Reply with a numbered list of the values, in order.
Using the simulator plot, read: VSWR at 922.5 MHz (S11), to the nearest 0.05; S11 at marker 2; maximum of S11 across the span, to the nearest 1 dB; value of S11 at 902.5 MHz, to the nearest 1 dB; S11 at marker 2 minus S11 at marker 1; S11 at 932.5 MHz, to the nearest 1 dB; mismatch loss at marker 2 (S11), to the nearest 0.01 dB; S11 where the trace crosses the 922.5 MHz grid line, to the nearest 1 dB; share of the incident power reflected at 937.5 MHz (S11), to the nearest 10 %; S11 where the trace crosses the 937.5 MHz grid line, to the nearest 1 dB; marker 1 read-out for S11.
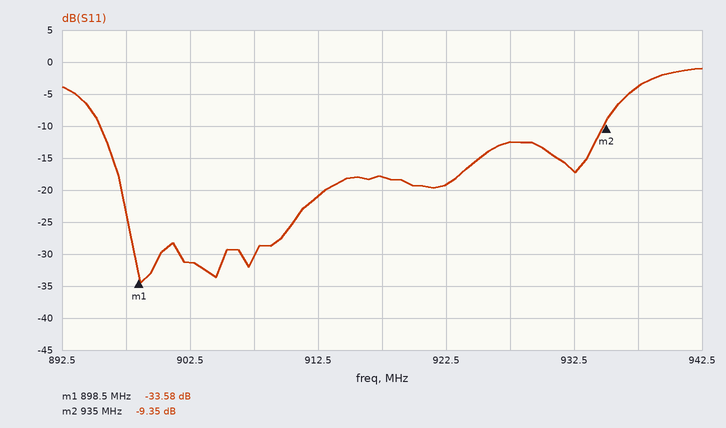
1. 1.25
2. -9.35 dB
3. -1 dB
4. -31 dB
5. 24.23 dB
6. -17 dB
7. 0.54 dB
8. -19 dB
9. 40 %
10. -4 dB
11. -33.58 dB
